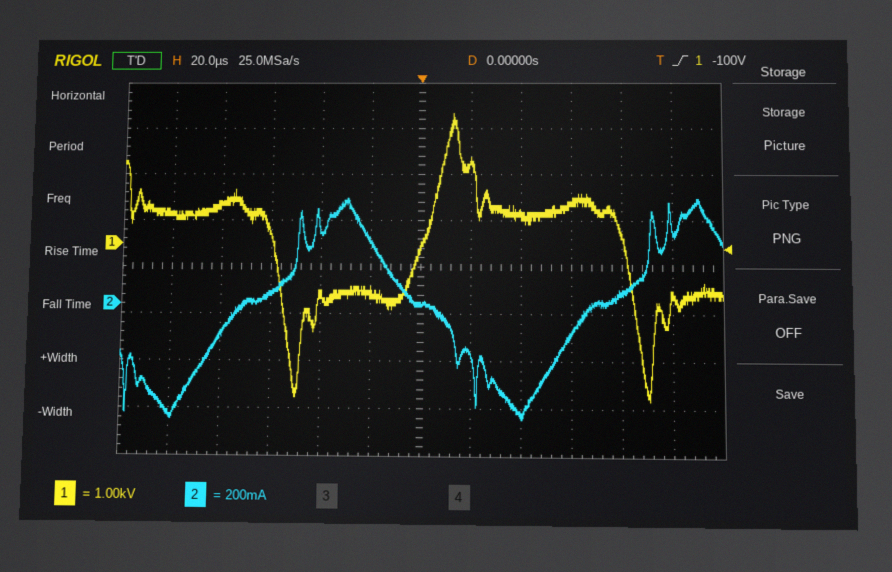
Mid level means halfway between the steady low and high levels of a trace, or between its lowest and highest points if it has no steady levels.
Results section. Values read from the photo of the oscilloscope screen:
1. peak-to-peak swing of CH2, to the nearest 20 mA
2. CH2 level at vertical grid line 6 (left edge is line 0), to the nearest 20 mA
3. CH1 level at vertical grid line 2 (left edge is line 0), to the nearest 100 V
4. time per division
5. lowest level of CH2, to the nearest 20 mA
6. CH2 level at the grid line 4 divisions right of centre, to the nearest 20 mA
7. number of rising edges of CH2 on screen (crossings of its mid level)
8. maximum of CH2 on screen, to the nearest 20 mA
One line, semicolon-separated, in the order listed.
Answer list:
940 mA; 0 mA; 800 V; 20 µs; -480 mA; 60 mA; 2; 460 mA
